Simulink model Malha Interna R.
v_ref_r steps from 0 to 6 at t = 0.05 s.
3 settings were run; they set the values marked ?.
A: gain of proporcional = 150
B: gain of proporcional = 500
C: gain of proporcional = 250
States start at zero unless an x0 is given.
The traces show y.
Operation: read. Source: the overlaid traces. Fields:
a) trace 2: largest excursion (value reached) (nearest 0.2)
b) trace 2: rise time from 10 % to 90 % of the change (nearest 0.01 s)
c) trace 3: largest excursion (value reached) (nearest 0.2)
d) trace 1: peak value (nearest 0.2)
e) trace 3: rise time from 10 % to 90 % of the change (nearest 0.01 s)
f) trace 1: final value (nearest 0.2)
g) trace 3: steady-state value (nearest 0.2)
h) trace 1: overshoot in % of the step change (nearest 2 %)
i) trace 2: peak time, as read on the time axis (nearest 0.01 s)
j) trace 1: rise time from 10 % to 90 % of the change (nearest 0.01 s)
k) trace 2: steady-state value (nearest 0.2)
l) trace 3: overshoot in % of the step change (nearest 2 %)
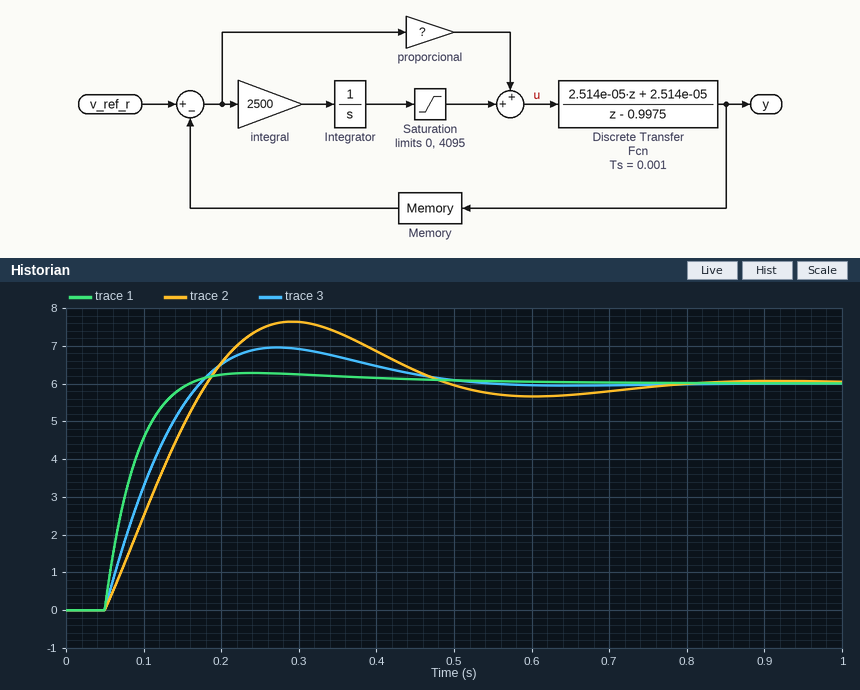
7.6
0.10 s
7.0
6.2
0.09 s
6.0
6.0
4 %
0.29 s
0.07 s
6.0
16 %
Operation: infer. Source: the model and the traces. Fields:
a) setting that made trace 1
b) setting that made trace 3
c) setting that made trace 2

B
C
A
